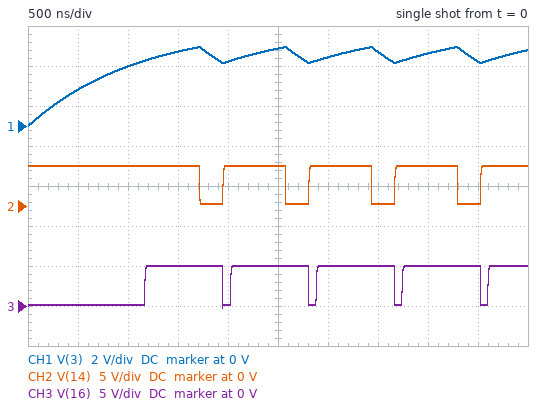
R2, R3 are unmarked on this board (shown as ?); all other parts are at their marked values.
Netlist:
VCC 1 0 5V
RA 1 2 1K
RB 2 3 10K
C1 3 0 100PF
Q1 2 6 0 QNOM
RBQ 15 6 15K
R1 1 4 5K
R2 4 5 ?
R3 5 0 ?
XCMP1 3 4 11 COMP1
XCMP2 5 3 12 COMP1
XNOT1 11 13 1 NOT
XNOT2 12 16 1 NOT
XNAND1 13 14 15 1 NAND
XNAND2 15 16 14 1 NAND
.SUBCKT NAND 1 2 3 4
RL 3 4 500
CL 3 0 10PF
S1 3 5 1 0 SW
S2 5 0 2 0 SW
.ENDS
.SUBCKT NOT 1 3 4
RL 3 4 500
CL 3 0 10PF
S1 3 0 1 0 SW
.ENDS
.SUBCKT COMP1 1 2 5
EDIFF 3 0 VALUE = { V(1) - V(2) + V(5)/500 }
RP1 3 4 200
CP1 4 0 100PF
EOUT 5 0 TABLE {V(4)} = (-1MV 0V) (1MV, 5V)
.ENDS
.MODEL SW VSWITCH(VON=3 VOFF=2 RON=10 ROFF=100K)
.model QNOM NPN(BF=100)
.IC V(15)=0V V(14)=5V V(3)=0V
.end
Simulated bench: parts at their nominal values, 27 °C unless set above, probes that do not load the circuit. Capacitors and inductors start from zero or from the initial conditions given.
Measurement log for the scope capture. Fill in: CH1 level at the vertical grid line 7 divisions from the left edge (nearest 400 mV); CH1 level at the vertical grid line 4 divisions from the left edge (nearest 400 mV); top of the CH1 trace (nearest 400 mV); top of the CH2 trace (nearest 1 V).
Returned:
3.6 V
3.2 V
4.0 V
5 V
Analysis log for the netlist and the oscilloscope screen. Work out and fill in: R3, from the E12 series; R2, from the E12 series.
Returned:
15 kΩ
3.3 kΩ
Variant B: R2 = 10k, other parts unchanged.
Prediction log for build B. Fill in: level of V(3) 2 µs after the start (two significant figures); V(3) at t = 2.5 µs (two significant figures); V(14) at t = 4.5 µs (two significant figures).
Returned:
4.2 V
2.6 V
5.0 V
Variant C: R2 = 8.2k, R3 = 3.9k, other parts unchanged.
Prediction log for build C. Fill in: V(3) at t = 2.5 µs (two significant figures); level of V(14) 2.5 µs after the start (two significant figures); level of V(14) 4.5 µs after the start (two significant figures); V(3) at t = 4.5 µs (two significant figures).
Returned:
1.2 V
190 mV
190 mV
1.6 V
